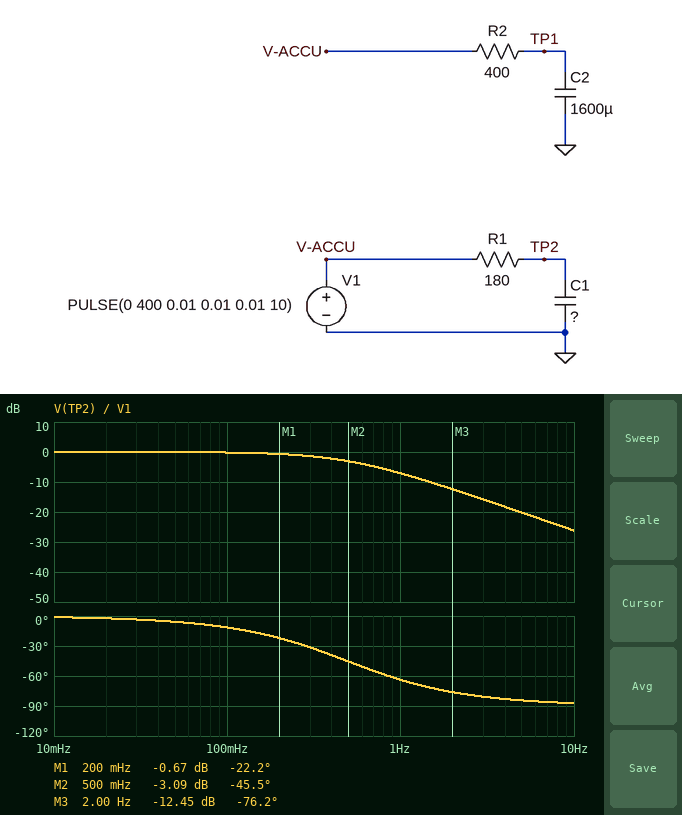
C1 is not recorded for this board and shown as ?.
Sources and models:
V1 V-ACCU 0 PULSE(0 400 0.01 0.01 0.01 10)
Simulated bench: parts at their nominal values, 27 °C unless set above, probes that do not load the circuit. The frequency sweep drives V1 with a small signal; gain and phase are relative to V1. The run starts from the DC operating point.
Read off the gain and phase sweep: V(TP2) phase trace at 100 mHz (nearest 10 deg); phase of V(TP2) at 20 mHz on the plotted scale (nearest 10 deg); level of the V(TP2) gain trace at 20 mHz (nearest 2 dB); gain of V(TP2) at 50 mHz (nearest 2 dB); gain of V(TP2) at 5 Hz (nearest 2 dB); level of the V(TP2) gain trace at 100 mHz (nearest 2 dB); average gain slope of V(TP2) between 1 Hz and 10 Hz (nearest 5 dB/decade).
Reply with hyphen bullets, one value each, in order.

- -10 deg
- 0 deg
- 0 dB
- 0 dB
- -20 dB
- 0 dB
- -20 dB/decade
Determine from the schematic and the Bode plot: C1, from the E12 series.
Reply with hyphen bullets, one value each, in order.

- 1.8 mF
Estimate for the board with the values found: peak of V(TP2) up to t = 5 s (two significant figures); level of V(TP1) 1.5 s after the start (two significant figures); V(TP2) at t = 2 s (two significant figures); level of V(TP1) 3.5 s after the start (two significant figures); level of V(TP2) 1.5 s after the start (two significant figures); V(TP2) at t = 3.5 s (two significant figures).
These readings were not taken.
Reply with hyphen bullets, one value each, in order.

- 400 V
- 360 V
- 400 V
- 400 V
- 400 V
- 400 V
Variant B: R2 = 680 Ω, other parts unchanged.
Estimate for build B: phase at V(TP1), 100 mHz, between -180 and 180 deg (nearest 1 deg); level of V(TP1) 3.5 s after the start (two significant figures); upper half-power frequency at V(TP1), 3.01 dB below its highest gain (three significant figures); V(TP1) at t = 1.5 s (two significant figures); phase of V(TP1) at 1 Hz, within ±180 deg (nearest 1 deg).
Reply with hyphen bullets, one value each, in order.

- -34 deg
- 380 V
- 146 mHz
- 300 V
- -82 deg
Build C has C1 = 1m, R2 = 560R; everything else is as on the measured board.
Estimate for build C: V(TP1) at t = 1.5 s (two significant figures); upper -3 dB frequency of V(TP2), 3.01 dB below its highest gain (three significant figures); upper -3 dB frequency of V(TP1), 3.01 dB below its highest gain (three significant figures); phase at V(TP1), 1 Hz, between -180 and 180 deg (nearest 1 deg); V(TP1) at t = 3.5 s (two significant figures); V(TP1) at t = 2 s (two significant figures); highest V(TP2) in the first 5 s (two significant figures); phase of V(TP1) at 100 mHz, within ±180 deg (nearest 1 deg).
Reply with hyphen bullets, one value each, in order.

- 320 V
- 884 mHz
- 178 mHz
- -80 deg
- 390 V
- 360 V
- 400 V
- -29 deg
